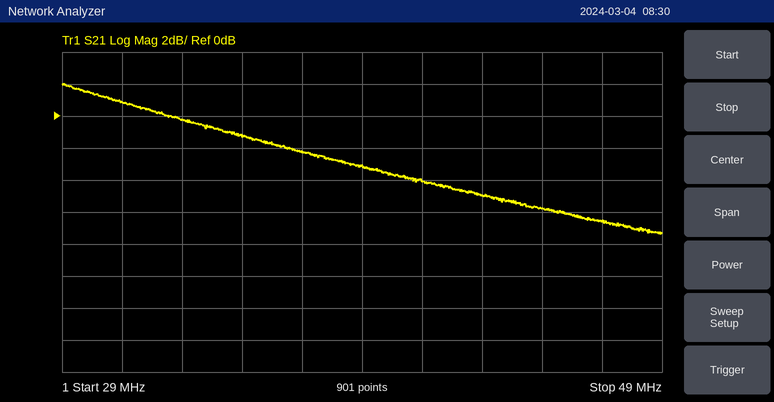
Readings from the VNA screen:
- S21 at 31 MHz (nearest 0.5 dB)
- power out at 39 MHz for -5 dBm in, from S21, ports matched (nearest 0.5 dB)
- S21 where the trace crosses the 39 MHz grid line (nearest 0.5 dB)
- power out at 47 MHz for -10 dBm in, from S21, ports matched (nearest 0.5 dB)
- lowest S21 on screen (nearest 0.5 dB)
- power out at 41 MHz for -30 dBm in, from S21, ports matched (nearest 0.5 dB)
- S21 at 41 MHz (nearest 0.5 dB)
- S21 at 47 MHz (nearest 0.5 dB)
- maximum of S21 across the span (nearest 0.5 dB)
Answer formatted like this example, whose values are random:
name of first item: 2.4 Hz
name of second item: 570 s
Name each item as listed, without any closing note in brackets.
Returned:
S21 at 31 MHz: 1.0 dB
power out at 39 MHz for -5 dBm in, from S21, ports matched: -8.0 dBm
S21 where the trace crosses the 39 MHz grid line: -3.0 dB
power out at 47 MHz for -10 dBm in, from S21, ports matched: -16.5 dBm
lowest S21 on screen: -7.5 dB
power out at 41 MHz for -30 dBm in, from S21, ports matched: -34.0 dBm
S21 at 41 MHz: -4.0 dB
S21 at 47 MHz: -6.5 dB
maximum of S21 across the span: 2.0 dB
